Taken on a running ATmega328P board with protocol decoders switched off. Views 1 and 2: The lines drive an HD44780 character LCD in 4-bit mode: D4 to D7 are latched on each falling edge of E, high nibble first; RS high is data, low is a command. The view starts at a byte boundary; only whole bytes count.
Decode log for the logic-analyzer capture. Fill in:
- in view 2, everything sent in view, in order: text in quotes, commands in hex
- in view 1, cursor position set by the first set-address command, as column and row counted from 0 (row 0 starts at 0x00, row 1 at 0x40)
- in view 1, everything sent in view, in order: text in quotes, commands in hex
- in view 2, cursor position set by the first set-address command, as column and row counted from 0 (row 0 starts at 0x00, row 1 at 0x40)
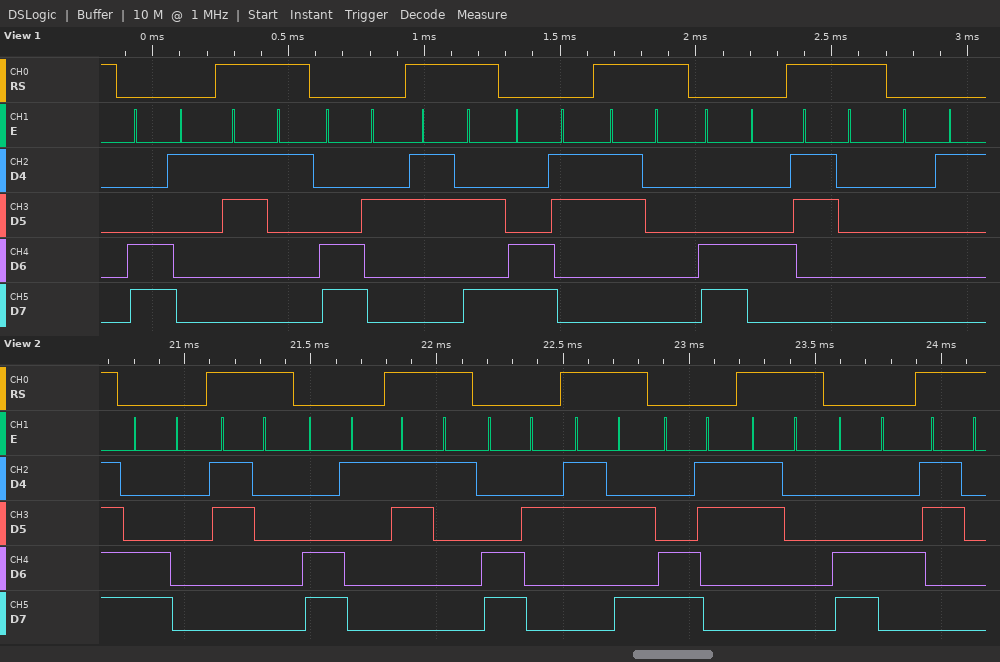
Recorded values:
0xC0 "0" 0xC1 "1" 0xC2 ":" 0xC3 "0" 0xC4 "0"
column 1, row 1
0xC1 "1" 0xC2 ":" 0xC3 "0" 0xC4 "0" 0x01
column 0, row 1
